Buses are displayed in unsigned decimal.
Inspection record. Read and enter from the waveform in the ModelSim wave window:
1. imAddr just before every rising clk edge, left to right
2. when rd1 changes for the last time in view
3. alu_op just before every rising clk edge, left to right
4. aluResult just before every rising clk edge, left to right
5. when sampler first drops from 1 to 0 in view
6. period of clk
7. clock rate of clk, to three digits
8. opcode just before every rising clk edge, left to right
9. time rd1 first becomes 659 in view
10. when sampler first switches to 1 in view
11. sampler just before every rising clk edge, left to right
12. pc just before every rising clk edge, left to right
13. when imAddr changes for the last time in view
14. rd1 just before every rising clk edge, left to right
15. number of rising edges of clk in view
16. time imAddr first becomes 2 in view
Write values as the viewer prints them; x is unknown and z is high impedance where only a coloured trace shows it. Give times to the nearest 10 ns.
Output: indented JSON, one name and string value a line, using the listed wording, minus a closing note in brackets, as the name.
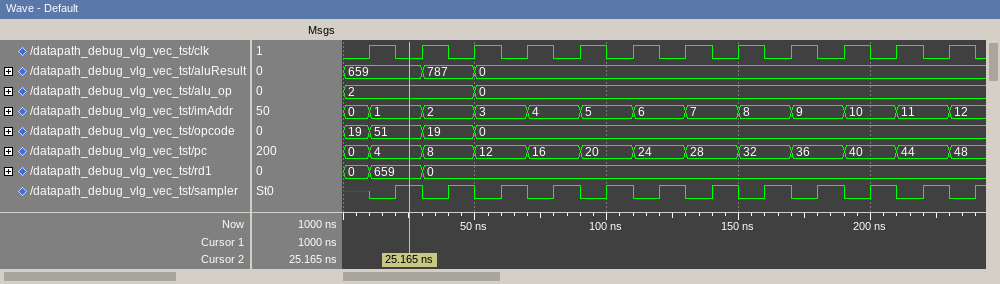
{
  "imAddr just before every rising clk edge, left to right": "0, 1, 2, 3, 4, 5, 6, 7, 8, 9, 10, 11",
  "when rd1 changes for the last time in view": "30 ns",
  "alu_op just before every rising clk edge, left to right": "2, 2, 2, 0, 0, 0, 0, 0, 0, 0, 0, 0",
  "aluResult just before every rising clk edge, left to right": "659, 659, 787, 0, 0, 0, 0, 0, 0, 0, 0, 0",
  "when sampler first drops from 1 to 0 in view": "30 ns",
  "period of clk": "20 ns",
  "clock rate of clk, to three digits": "50.0 MHz",
  "opcode just before every rising clk edge, left to right": "19, 51, 19, 0, 0, 0, 0, 0, 0, 0, 0, 0",
  "time rd1 first becomes 659 in view": "10 ns",
  "when sampler first switches to 1 in view": "20 ns",
  "sampler just before every rising clk edge, left to right": "x 1 1 1 1 1 1 1 1 1 1 1",
  "pc just before every rising clk edge, left to right": "0, 4, 8, 12, 16, 20, 24, 28, 32, 36, 40, 44",
  "when imAddr changes for the last time in view": "230 ns",
  "rd1 just before every rising clk edge, left to right": "0, 659, 0, 0, 0, 0, 0, 0, 0, 0, 0, 0",
  "number of rising edges of clk in view": "12",
  "time imAddr first becomes 2 in view": "30 ns"
}
